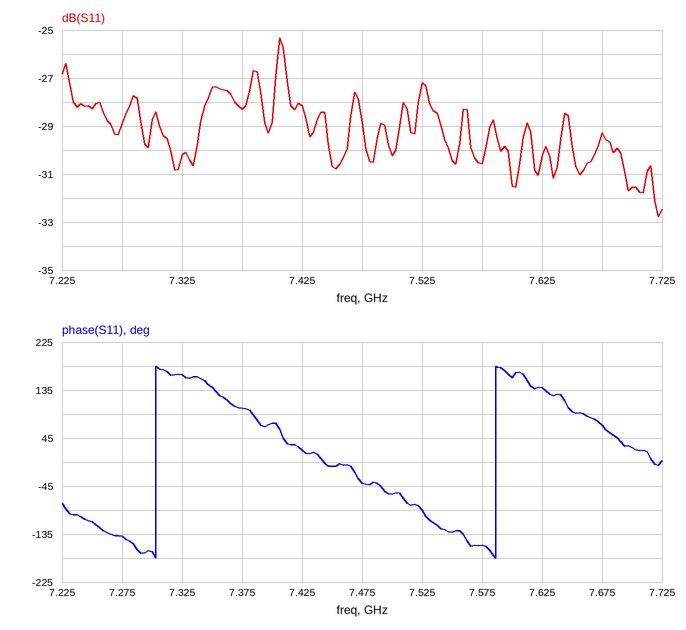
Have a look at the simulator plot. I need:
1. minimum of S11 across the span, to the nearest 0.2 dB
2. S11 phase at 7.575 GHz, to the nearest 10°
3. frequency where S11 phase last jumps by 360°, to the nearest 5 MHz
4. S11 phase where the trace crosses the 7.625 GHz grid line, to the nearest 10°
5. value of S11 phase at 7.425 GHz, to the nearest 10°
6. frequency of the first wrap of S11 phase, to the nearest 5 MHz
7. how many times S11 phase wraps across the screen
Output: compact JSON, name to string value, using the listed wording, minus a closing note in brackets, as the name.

{"minimum of S11 across the span, to the nearest 0.2 dB": "-32.8 dB", "S11 phase at 7.575 GHz, to the nearest 10°": "-160°", "frequency where S11 phase last jumps by 360°, to the nearest 5 MHz": "7.585 GHz", "S11 phase where the trace crosses the 7.625 GHz grid line, to the nearest 10°": "140°", "value of S11 phase at 7.425 GHz, to the nearest 10°": "20°", "frequency of the first wrap of S11 phase, to the nearest 5 MHz": "7.305 GHz", "how many times S11 phase wraps across the screen": "2"}
